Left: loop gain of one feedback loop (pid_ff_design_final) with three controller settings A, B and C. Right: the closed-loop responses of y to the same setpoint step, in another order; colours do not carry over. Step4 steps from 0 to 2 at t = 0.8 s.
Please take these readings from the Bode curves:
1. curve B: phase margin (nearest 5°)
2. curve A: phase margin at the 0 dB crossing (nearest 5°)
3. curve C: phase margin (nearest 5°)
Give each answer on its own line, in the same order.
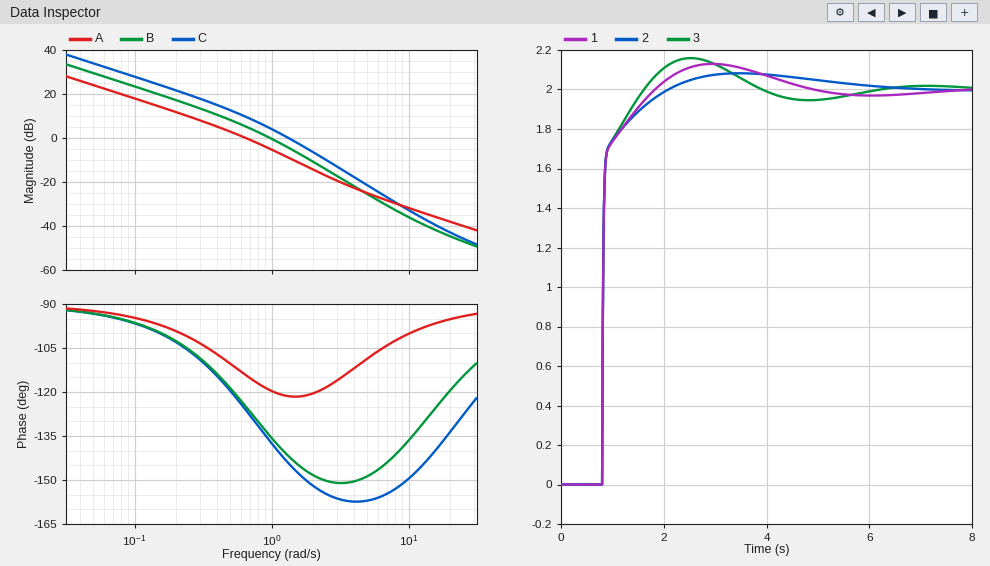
45°
65°
35°
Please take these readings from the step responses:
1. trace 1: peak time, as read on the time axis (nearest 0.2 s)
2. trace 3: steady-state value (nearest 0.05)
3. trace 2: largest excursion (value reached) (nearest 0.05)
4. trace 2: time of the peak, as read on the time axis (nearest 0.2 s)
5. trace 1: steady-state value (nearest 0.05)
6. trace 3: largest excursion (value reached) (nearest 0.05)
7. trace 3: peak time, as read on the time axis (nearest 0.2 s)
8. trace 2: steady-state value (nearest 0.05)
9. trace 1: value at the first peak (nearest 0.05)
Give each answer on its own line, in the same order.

3.0 s
2.00
2.10
3.4 s
2.00
2.15
2.6 s
2.00
2.15
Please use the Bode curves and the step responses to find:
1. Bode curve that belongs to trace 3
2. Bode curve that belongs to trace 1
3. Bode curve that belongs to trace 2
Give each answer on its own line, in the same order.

C
B
A
